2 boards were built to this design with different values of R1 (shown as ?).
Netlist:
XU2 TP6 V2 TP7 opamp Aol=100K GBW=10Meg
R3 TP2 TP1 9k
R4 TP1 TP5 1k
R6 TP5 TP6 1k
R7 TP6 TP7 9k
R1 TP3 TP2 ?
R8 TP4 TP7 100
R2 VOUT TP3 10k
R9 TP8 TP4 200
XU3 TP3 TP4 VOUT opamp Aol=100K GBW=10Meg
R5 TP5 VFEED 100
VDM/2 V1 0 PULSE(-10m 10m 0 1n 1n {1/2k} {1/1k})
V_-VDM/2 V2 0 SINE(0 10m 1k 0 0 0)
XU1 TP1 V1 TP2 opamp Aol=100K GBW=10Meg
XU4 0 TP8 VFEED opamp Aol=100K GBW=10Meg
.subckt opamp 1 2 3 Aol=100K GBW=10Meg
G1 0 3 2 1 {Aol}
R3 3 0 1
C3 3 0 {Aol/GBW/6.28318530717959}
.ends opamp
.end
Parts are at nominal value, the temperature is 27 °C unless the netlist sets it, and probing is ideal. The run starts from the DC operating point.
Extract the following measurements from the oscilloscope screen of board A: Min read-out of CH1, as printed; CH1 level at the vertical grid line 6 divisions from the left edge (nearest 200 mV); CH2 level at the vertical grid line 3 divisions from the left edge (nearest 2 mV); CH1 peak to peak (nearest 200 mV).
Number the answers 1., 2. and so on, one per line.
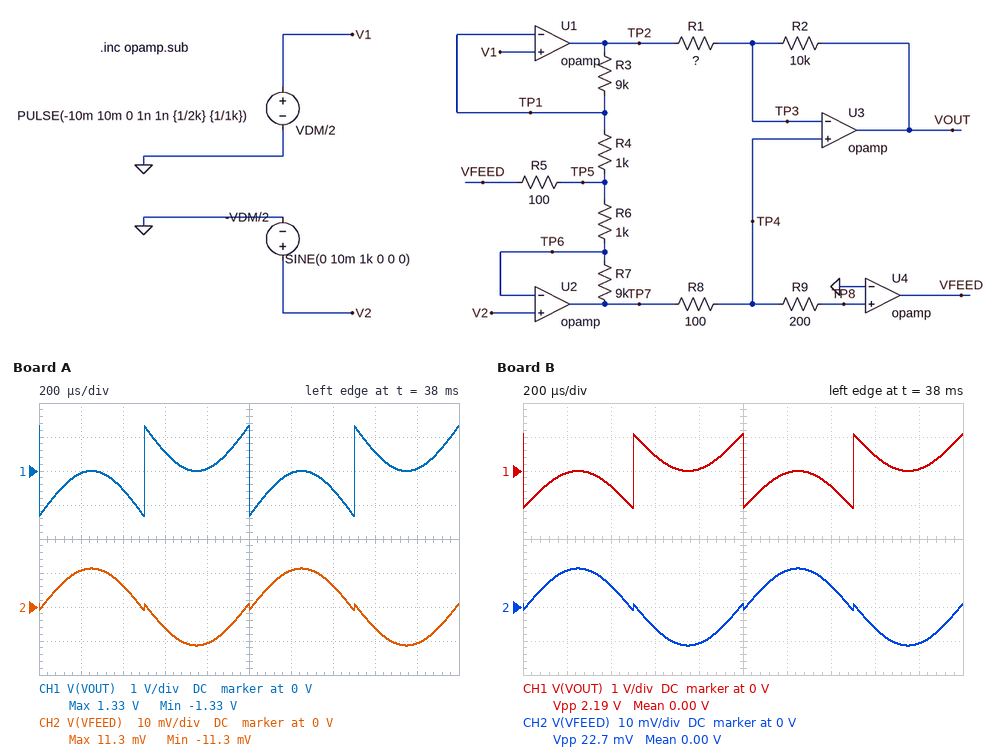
1. -1.33 V
2. 0 V
3. -6 mV
4. 2.6 V
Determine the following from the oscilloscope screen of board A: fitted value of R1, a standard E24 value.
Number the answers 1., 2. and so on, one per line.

1. 750 Ω
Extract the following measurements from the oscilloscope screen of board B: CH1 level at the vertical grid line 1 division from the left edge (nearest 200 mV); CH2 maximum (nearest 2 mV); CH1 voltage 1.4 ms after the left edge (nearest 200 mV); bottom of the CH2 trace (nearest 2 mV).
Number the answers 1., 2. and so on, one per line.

1. 0 V
2. 12 mV
3. -400 mV
4. -12 mV
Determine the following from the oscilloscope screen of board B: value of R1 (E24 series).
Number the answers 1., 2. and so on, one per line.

1. 910 Ω
